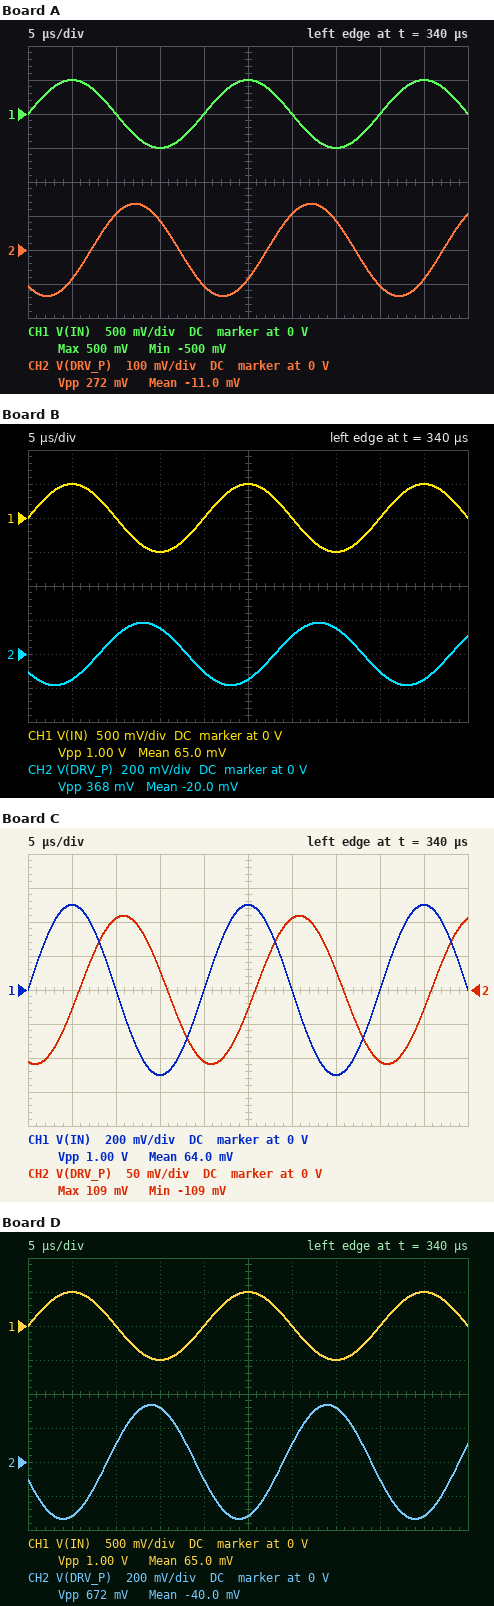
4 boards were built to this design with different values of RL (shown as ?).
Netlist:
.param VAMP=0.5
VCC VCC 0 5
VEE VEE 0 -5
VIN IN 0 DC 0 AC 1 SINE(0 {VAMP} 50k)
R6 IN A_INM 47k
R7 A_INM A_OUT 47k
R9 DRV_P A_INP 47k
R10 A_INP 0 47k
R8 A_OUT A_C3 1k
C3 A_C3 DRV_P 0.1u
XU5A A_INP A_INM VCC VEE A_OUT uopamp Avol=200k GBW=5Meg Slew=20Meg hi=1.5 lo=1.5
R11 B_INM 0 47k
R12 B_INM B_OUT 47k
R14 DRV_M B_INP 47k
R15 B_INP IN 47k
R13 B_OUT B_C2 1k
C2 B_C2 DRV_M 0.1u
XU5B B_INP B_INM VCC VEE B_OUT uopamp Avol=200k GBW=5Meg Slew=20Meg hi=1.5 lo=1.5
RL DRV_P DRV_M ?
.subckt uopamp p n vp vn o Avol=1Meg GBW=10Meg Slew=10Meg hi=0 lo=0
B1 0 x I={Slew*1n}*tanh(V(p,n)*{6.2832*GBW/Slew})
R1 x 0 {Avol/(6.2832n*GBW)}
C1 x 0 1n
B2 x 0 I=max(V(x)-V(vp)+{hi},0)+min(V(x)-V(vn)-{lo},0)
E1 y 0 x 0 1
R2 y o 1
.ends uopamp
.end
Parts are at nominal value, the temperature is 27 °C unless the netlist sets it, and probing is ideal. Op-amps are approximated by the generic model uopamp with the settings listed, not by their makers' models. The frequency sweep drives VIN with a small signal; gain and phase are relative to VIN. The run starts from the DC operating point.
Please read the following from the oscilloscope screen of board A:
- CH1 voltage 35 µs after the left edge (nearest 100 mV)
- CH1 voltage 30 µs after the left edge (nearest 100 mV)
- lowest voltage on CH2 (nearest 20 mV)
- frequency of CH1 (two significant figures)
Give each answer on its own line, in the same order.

-500 mV
0 V
-140 mV
50 kHz
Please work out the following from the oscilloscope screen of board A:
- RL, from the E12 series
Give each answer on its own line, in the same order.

560 Ω
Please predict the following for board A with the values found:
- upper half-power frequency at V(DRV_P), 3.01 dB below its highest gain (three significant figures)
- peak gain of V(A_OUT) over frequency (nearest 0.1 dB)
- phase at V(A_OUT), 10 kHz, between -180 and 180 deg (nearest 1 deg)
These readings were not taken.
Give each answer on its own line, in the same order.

2.65 kHz
2.0 dB
-165 deg
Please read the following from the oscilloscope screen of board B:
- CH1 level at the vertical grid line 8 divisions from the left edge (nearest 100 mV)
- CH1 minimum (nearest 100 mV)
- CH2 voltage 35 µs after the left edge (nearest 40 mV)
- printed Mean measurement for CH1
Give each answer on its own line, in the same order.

0 V
-500 mV
160 mV
65.0 mV
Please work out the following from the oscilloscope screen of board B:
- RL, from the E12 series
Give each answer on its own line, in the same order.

820 Ω
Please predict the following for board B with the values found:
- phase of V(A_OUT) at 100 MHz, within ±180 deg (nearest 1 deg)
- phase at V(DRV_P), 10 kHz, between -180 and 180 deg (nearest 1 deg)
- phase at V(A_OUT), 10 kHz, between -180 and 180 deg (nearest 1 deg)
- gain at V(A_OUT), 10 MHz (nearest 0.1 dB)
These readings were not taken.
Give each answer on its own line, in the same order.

91 deg
-76 deg
-166 deg
-12.2 dB
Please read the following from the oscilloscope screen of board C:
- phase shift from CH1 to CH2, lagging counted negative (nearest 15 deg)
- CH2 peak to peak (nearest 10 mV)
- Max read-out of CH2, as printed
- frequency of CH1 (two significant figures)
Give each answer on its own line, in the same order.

-105 deg
220 mV
109 mV
50 kHz
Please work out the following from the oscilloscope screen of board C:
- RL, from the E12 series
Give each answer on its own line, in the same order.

330 Ω
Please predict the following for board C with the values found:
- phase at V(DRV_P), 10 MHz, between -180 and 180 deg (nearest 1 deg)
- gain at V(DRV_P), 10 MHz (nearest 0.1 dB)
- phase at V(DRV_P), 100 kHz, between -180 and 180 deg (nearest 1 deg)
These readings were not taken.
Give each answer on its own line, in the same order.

95 deg
-29.7 dB
-138 deg
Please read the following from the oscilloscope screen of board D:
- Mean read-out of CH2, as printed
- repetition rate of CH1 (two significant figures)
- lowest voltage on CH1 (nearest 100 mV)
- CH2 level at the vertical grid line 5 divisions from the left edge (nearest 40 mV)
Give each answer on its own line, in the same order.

-40.0 mV
50 kHz
-500 mV
-320 mV
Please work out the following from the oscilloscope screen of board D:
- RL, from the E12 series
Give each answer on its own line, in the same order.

1.5 kΩ
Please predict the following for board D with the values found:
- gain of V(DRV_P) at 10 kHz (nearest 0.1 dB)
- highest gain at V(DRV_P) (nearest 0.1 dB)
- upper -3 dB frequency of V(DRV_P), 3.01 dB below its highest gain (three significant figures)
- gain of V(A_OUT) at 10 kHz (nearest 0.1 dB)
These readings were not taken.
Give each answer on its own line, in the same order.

-8.0 dB
-2.8 dB
1.48 MHz
2.3 dB
